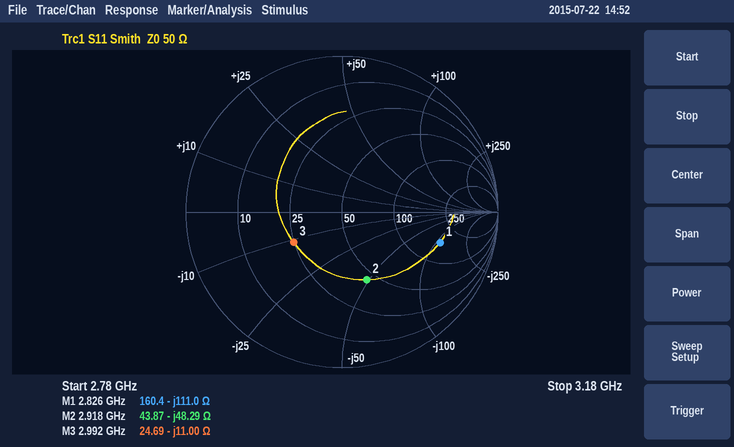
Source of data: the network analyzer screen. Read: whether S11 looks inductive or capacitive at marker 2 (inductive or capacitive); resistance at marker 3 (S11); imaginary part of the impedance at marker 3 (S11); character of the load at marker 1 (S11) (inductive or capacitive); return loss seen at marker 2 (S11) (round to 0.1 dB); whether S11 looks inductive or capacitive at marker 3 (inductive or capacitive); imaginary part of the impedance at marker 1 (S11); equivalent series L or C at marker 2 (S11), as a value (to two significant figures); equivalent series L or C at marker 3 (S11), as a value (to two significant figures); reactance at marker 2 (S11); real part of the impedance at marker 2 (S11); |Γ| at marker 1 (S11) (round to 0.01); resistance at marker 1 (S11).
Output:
capacitive
24.69 Ω
-11.00 Ω
capacitive
6.7 dB
capacitive
-111.0 Ω
1.1 pF
4.8 pF
-48.29 Ω
43.87 Ω
0.66
160.4 Ω
